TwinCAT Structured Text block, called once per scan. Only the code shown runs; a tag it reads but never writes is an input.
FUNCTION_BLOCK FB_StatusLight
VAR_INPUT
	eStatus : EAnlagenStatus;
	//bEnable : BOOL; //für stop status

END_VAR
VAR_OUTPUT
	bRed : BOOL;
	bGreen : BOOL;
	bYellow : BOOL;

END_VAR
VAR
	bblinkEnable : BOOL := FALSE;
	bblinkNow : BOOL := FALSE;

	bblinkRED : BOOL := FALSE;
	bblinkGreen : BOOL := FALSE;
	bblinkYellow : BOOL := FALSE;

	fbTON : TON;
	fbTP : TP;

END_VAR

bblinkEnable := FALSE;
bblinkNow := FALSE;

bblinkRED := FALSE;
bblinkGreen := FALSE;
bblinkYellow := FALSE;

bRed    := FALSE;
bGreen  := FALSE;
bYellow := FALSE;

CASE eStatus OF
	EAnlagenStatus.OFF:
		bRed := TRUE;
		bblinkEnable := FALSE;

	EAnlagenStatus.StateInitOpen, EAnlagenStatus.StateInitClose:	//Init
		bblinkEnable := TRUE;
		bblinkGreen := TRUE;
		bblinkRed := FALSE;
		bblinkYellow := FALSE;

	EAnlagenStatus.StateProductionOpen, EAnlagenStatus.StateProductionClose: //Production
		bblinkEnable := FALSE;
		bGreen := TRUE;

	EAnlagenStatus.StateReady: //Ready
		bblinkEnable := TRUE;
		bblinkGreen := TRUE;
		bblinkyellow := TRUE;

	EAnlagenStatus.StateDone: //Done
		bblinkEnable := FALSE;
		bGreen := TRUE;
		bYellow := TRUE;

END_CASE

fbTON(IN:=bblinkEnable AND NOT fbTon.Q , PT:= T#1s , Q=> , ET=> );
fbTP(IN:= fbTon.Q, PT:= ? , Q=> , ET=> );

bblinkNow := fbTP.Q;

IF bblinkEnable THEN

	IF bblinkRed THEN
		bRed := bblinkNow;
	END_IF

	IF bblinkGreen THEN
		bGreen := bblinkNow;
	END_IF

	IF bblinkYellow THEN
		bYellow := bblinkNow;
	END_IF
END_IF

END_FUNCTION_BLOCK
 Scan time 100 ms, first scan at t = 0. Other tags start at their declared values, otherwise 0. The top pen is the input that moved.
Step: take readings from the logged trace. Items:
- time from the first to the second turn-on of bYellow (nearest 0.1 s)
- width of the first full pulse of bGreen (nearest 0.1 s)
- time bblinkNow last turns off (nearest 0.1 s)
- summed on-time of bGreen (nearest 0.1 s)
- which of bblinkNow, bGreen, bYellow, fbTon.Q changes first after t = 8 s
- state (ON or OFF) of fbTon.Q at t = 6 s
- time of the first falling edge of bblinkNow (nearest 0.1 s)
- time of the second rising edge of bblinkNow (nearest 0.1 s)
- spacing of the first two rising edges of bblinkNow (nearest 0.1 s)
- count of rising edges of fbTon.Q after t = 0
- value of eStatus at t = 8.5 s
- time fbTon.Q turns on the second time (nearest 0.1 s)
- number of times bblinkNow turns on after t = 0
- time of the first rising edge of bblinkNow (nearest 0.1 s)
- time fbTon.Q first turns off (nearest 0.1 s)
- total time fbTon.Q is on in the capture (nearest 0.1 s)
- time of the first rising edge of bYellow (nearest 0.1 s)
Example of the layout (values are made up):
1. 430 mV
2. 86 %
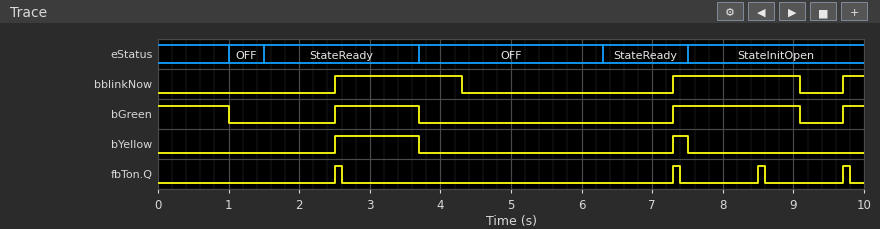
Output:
1. 4.8 s
2. 1.2 s
3. 9.1 s
4. 4.3 s
5. fbTon.Q
6. OFF
7. 4.3 s
8. 7.3 s
9. 4.8 s
10. 4
11. StateInitOpen
12. 7.3 s
13. 3
14. 2.5 s
15. 2.6 s
16. 0.4 s
17. 2.5 s
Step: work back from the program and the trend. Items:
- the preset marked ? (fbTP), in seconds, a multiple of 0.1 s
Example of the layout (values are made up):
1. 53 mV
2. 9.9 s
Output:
1. 1.8 s
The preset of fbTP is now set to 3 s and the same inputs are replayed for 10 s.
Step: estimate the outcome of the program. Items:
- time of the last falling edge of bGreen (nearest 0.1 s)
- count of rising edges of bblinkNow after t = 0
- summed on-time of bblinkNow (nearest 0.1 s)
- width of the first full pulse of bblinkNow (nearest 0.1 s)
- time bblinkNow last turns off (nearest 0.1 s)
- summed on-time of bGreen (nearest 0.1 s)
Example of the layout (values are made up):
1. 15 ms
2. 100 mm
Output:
1. 3.7 s
2. 2
3. 5.7 s
4. 3.0 s
5. 5.5 s
6. 4.9 s
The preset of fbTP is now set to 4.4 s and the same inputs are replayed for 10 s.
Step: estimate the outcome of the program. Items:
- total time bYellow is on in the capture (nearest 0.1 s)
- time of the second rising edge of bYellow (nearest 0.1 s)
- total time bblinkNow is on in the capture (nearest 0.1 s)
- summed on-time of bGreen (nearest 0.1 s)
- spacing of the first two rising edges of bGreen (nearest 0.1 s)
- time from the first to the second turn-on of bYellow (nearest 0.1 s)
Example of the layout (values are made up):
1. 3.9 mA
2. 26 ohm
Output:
1. 2.0 s
2. 6.3 s
3. 7.1 s
4. 5.5 s
5. 3.8 s
6. 3.8 s
